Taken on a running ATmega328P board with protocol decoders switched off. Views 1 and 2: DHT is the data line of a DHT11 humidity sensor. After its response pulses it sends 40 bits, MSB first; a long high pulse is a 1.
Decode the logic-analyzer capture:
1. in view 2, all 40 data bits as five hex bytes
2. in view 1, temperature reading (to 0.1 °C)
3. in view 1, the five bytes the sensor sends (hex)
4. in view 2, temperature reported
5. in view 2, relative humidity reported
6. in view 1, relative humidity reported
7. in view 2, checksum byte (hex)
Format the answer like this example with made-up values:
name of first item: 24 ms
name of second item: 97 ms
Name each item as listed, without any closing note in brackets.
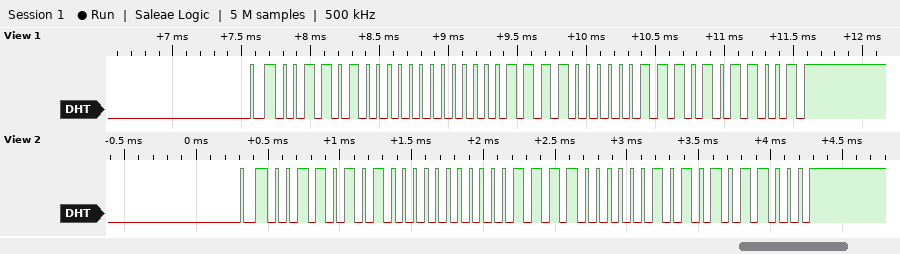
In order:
in view 2, all 40 data bits as five hex bytes: 35 00 1E 05 58
in view 1, temperature reading: 30.7 °C
in view 1, the five bytes the sensor sends: 34 00 1E 07 59
in view 2, temperature reported: 30.5 °C
in view 2, relative humidity reported: 53 %
in view 1, relative humidity reported: 52 %
in view 2, checksum byte: 0x58
